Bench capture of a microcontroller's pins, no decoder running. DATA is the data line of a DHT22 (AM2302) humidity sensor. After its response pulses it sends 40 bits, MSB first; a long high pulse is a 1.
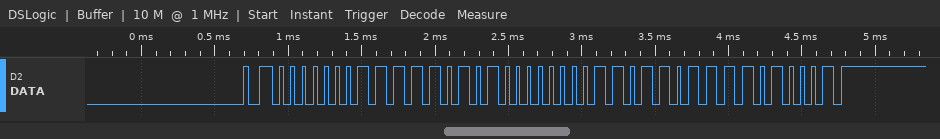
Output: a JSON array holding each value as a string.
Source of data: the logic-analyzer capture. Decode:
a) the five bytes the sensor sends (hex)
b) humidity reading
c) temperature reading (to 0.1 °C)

["01 F5 00 DB D1", "50.1 %", "21.9 °C"]
